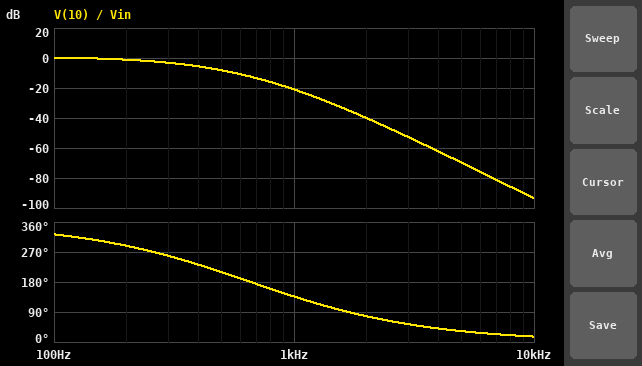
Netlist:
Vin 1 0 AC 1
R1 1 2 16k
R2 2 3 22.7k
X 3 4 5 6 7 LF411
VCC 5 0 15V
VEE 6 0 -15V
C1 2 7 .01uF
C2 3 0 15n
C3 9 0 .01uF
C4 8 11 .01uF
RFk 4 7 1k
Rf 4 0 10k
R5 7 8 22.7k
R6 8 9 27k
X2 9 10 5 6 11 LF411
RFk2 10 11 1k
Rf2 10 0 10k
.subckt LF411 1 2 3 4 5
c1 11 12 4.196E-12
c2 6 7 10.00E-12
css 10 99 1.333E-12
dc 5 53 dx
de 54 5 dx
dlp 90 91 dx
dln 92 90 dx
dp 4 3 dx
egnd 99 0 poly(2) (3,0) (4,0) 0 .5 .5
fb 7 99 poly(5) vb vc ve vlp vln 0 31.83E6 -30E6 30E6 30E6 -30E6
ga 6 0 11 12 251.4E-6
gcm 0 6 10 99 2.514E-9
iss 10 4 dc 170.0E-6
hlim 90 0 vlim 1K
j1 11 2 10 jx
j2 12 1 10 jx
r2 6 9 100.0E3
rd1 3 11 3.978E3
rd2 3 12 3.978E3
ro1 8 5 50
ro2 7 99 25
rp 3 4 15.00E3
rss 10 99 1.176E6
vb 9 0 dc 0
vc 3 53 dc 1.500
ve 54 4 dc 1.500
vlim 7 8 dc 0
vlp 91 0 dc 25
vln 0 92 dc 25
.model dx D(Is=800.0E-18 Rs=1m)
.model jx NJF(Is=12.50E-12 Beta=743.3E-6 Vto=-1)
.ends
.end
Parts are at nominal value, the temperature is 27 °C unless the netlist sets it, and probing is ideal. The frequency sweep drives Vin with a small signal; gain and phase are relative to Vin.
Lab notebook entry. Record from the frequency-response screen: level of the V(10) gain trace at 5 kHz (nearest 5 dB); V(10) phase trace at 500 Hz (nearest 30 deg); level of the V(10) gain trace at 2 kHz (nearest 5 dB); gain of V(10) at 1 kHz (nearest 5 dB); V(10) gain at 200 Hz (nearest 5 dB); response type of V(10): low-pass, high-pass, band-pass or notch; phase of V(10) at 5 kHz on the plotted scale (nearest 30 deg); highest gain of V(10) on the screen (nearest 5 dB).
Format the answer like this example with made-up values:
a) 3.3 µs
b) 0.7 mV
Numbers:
a) -70 dB
b) 210 deg
c) -40 dB
d) -20 dB
e) 0 dB
f) low-pass
g) 30 deg
h) 0 dB
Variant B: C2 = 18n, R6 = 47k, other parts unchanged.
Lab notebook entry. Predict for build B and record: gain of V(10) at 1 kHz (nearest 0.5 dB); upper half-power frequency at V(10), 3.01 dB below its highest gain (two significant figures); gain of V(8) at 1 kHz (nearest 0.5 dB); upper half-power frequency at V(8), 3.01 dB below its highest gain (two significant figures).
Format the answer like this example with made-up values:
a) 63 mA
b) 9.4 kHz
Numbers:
a) -27.0 dB
b) 190 Hz
c) -17.0 dB
d) 250 Hz
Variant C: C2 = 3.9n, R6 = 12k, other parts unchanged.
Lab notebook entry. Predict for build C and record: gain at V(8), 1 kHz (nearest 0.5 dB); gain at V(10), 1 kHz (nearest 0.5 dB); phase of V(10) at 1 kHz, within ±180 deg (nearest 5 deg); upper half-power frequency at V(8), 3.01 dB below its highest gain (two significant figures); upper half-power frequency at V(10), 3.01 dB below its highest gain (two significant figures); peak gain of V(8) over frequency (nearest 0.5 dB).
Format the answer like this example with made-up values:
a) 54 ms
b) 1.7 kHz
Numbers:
a) -3.0 dB
b) -5.0 dB
c) -155 deg
d) 890 Hz
e) 700 Hz
f) 1.0 dB
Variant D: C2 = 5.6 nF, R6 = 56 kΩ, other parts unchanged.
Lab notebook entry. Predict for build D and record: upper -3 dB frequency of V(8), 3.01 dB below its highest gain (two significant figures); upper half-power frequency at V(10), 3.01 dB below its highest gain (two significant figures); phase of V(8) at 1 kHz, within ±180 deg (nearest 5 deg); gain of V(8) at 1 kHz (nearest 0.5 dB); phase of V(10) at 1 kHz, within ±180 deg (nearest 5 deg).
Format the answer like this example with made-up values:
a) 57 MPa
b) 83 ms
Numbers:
a) 660 Hz
b) 260 Hz
c) -135 deg
d) -6.0 dB
e) 150 deg
